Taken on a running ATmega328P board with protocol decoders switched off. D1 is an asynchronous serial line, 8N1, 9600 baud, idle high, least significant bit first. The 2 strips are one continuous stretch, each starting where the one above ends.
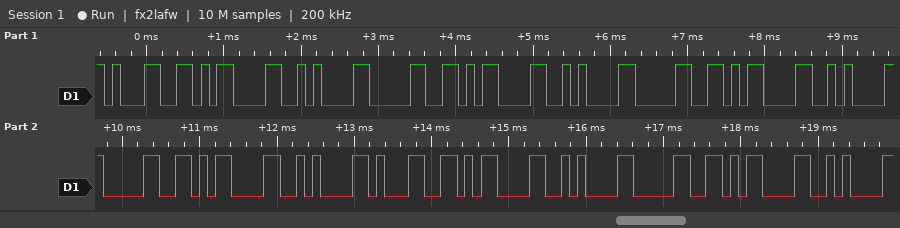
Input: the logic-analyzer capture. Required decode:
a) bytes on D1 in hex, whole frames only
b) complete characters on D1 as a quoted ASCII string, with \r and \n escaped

31 0D 0A 30 0D 0A 30 0D 0A 30 0D 0A 31 0D 0A 30 0D 0A
"1\r\n0\r\n0\r\n0\r\n1\r\n0\r\n"
